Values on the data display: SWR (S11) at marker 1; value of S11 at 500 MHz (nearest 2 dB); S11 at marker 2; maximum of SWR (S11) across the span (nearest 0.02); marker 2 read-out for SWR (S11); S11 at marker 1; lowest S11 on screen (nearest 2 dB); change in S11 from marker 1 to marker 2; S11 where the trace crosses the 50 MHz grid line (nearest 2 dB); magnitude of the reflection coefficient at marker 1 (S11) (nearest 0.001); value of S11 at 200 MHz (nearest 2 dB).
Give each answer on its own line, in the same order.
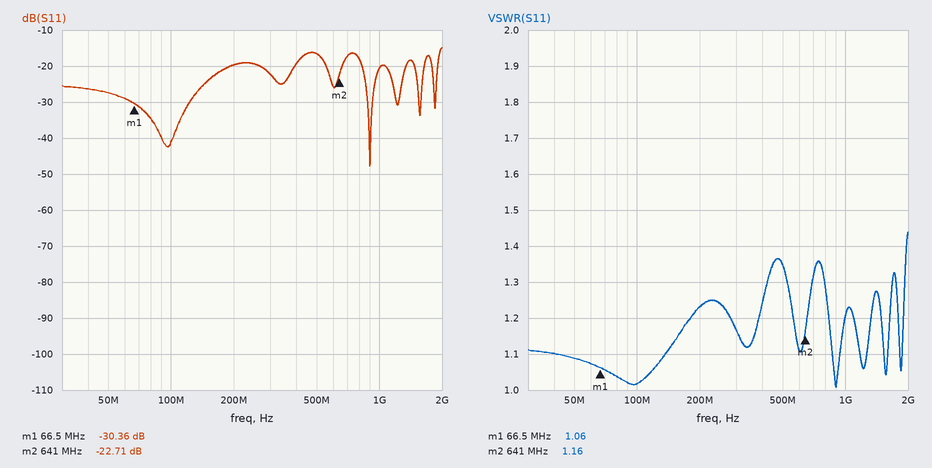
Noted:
1.06
-16 dB
-22.71 dB
1.44
1.16
-30.36 dB
-48 dB
7.65 dB
-28 dB
0.030
-20 dB
